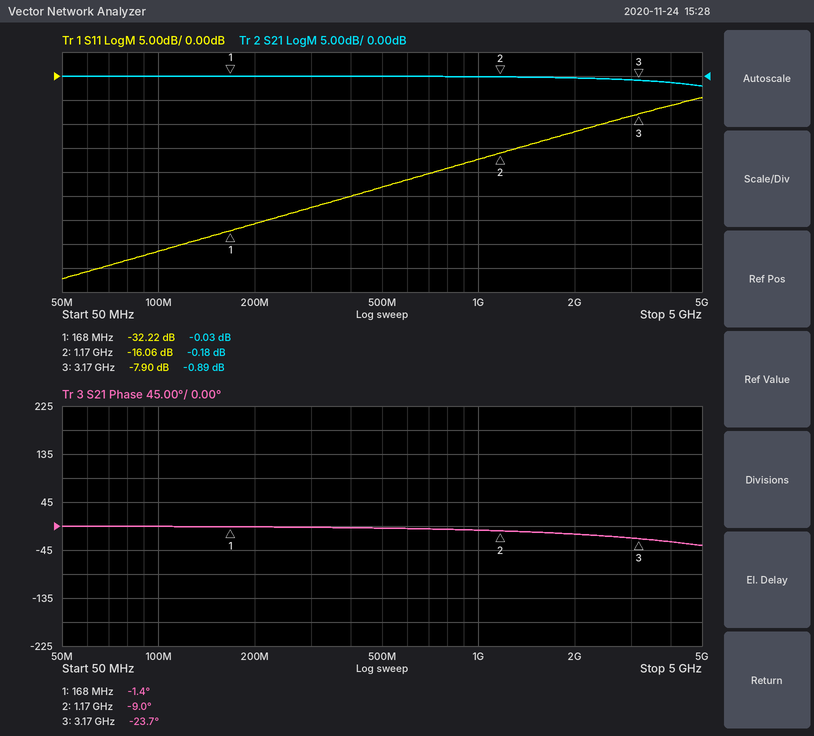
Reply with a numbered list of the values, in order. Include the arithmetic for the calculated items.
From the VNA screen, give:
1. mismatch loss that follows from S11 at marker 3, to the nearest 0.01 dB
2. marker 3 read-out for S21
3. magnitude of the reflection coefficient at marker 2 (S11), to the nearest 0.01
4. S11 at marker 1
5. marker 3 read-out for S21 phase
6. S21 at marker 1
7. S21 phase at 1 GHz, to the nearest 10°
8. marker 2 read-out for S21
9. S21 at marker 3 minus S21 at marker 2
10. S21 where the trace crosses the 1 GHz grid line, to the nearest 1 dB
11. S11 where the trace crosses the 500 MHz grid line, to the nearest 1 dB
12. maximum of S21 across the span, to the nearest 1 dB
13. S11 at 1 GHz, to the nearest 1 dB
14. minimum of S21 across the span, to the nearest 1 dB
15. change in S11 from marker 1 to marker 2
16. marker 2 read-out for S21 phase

1. −10 log10(1 − 10^(-7.9/10)) ≈ 0.77 dB
2. -0.89 dB
3. 10^(-16.06/20) ≈ 0.16
4. -32.22 dB
5. -23.7°
6. -0.03 dB
7. -10°
8. -0.18 dB
9. -0.89 − (-0.18) = -0.71 dB
10. 0 dB
11. -23 dB
12. 0 dB
13. -17 dB
14. -2 dB
15. -16.06 − (-32.22) = 16.16 dB
16. -9.0°
